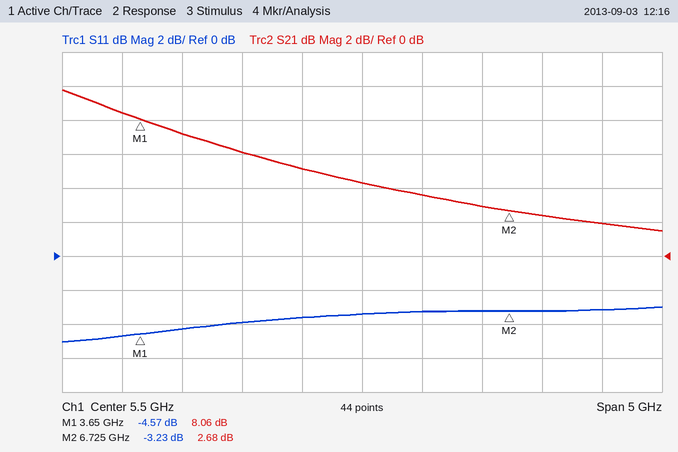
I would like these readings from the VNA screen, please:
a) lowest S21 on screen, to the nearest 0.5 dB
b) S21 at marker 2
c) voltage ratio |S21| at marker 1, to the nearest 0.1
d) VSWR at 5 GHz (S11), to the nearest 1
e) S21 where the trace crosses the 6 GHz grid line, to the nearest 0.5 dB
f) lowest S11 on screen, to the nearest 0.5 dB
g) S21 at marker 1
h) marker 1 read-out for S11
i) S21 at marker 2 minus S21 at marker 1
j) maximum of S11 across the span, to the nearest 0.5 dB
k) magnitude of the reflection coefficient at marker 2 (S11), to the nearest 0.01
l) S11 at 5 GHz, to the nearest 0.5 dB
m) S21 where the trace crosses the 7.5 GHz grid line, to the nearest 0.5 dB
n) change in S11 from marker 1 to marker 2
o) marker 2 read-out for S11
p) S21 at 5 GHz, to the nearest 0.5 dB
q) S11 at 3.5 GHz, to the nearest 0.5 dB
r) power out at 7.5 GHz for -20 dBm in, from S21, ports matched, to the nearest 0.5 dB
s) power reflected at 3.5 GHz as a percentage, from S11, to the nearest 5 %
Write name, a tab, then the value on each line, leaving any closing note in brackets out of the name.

lowest S21 on screen, to the nearest 0.5 dB	1.5 dB
S21 at marker 2	2.68 dB
voltage ratio |S21| at marker 1, to the nearest 0.1	2.5
VSWR at 5 GHz (S11), to the nearest 1	5
S21 where the trace crosses the 6 GHz grid line, to the nearest 0.5 dB	3.5 dB
lowest S11 on screen, to the nearest 0.5 dB	-5.0 dB
S21 at marker 1	8.06 dB
marker 1 read-out for S11	-4.57 dB
S21 at marker 2 minus S21 at marker 1	-5.38 dB
maximum of S11 across the span, to the nearest 0.5 dB	-3.0 dB
magnitude of the reflection coefficient at marker 2 (S11), to the nearest 0.01	0.69
S11 at 5 GHz, to the nearest 0.5 dB	-3.5 dB
S21 where the trace crosses the 7.5 GHz grid line, to the nearest 0.5 dB	2.0 dB
change in S11 from marker 1 to marker 2	1.34 dB
marker 2 read-out for S11	-3.23 dB
S21 at 5 GHz, to the nearest 0.5 dB	5.0 dB
S11 at 3.5 GHz, to the nearest 0.5 dB	-4.5 dB
power out at 7.5 GHz for -20 dBm in, from S21, ports matched, to the nearest 0.5 dB	-18.0 dBm
power reflected at 3.5 GHz as a percentage, from S11, to the nearest 5 %	35 %
